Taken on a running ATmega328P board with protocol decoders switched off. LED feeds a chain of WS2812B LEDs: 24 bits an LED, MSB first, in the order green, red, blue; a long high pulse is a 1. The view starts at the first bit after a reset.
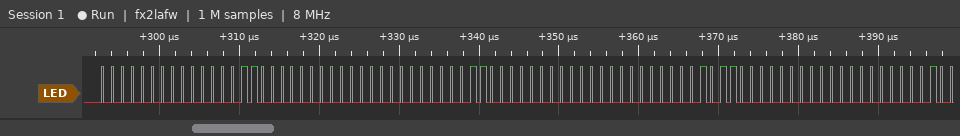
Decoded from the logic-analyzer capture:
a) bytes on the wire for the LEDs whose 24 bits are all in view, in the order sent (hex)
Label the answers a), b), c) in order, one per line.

a) 00 03 00 00 06 00 00 0B 00
